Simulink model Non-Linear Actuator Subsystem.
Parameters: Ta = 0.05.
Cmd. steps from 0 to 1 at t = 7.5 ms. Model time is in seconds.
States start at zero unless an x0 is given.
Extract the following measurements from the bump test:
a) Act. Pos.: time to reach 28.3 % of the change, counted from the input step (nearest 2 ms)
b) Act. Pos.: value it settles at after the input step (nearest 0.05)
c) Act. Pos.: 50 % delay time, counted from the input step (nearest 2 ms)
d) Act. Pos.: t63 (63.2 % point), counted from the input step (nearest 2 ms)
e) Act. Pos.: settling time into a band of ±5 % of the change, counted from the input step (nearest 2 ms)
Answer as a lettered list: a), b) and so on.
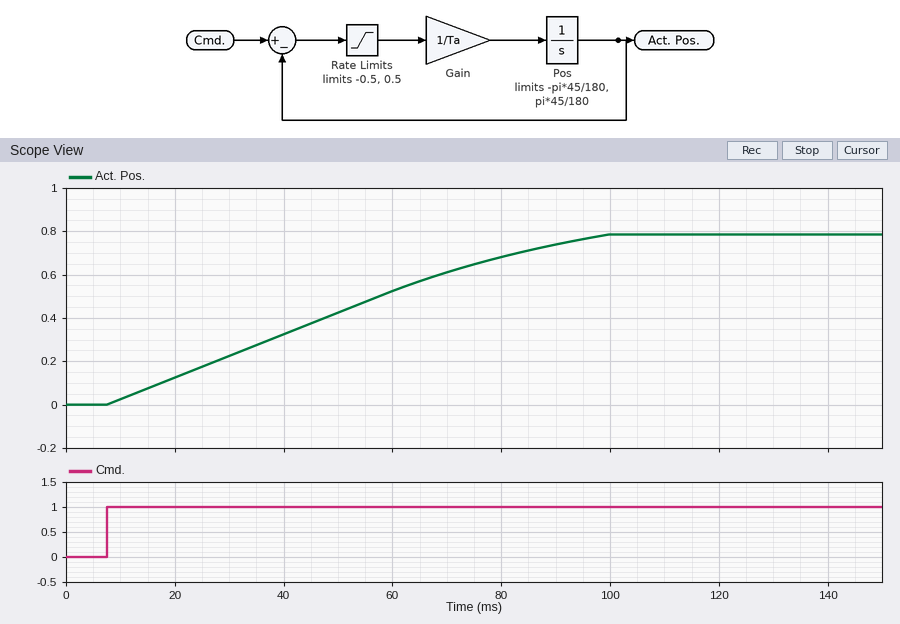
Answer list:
a) 22 ms
b) 0.80
c) 40 ms
d) 50 ms
e) 84 ms
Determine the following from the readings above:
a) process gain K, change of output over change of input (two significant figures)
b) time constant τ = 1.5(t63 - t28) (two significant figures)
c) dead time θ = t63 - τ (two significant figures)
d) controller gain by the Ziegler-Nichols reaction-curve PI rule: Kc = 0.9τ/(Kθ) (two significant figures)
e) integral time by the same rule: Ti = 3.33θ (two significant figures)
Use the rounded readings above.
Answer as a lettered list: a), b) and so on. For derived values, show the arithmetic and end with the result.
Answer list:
a) (0.8 - 0) / 1 = 0.80
b) 1.5 × (50 - 22) = 42 ms
c) 50 - 42 = 8.0 ms
d) 0.9 × 42 / (0.8 × 8) = 5.9
e) 3.33 × 8 = 27 ms
